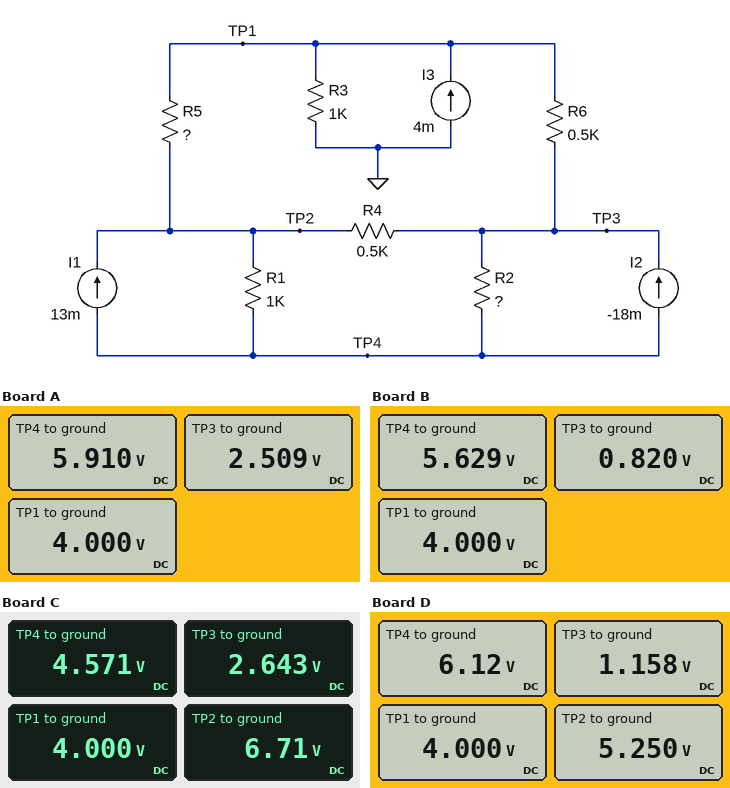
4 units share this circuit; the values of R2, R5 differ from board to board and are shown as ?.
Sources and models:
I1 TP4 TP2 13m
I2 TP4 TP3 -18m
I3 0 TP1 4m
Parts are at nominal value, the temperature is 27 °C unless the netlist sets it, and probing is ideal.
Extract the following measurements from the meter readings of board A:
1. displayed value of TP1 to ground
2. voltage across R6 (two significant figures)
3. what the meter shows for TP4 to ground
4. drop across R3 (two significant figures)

4.000 V
1.5 V
5.910 V
4.0 V
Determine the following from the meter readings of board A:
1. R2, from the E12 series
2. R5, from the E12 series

560 Ω
1 kΩ
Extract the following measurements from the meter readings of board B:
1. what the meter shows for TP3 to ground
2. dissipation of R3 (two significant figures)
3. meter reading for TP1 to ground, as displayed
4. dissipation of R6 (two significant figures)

0.820 V
16 mW
4.000 V
20 mW
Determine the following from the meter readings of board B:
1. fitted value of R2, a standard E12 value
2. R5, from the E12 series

1.2 kΩ
100 Ω
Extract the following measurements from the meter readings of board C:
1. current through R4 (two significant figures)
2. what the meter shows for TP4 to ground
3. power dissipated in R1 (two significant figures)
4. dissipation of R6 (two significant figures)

8.1 mA
4.571 V
4.6 mW
3.7 mW
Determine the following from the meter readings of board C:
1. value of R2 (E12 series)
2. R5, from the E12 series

270 Ω
1 kΩ
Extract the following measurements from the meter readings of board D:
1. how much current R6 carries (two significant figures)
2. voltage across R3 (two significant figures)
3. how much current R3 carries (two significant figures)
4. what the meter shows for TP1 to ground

5.7 mA
4.0 V
4.0 mA
4.000 V
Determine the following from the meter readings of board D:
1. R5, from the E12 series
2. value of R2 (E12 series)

220 Ω
1.2 kΩ
